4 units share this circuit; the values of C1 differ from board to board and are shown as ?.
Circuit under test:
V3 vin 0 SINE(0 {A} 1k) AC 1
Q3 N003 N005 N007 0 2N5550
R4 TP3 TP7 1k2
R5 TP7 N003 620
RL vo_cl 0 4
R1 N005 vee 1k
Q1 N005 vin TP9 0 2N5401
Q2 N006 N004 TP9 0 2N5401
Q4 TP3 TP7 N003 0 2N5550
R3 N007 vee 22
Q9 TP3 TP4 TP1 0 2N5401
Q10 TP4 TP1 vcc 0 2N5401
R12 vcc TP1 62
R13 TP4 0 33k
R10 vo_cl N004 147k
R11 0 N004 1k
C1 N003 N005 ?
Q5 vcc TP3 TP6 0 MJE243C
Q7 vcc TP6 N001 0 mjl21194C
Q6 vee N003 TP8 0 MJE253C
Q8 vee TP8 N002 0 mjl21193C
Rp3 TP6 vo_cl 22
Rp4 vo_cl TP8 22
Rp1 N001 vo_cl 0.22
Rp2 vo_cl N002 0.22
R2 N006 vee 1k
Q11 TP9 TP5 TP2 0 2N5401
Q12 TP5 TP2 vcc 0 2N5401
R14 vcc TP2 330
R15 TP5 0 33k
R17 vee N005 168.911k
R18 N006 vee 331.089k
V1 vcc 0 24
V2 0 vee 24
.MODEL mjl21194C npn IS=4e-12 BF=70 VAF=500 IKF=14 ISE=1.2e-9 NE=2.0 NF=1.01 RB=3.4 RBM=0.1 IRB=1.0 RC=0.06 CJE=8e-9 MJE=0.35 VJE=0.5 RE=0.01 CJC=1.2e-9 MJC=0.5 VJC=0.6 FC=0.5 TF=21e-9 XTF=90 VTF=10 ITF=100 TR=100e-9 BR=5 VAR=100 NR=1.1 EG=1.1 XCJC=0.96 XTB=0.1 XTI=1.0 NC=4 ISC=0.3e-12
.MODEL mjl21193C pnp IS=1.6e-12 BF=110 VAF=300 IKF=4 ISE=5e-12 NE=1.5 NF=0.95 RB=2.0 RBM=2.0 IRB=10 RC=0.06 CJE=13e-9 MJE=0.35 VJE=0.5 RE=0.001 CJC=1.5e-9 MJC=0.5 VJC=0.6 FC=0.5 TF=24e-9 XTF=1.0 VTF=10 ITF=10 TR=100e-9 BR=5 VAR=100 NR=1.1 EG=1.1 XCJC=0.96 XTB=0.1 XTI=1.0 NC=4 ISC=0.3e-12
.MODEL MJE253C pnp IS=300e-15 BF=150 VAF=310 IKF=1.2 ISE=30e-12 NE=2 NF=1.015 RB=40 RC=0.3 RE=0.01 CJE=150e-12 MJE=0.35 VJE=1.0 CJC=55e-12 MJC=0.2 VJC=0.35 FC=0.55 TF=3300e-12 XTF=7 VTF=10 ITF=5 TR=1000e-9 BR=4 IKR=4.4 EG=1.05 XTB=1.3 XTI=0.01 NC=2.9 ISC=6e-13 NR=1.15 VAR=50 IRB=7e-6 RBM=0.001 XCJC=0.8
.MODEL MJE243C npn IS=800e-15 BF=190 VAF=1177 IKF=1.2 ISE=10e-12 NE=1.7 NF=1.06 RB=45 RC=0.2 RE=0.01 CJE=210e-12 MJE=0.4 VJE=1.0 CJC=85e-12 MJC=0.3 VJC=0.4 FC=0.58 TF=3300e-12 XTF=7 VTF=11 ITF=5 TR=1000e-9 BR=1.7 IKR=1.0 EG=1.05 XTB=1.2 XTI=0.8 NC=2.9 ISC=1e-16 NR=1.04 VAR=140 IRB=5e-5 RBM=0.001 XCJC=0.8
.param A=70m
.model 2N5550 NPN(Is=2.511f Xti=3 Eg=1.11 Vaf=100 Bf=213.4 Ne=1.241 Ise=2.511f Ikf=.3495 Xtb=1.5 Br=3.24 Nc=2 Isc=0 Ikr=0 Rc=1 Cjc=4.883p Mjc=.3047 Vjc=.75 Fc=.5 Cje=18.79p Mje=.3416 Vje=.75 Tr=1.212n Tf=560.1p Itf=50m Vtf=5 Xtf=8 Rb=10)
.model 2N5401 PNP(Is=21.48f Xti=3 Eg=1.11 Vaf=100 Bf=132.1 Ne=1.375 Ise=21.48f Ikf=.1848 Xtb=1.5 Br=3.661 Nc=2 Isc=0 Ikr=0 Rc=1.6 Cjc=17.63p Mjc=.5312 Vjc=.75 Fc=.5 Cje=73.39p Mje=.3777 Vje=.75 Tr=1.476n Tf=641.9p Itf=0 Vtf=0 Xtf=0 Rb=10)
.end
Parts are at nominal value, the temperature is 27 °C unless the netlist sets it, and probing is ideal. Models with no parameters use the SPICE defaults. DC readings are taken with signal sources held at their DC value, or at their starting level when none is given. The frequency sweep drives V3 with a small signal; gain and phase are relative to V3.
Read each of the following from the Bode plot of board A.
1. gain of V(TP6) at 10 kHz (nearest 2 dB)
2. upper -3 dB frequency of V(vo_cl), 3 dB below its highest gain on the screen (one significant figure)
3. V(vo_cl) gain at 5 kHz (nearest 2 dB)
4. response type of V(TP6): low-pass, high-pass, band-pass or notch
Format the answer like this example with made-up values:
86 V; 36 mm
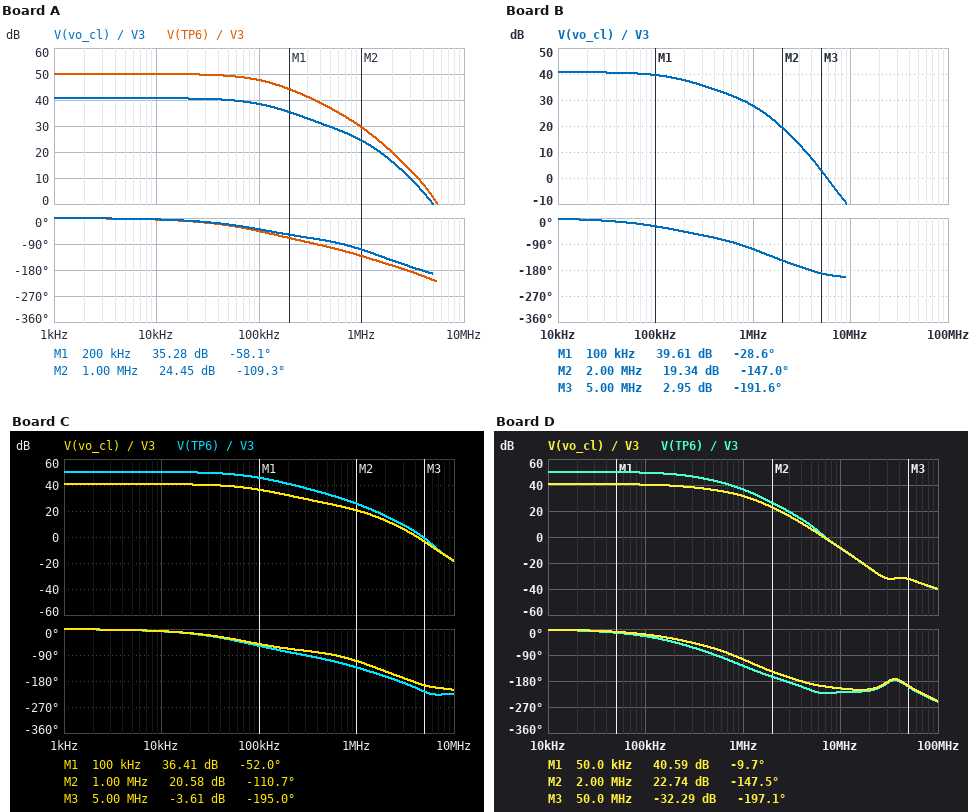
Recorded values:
50 dB; 100 kHz; 40 dB; low-pass
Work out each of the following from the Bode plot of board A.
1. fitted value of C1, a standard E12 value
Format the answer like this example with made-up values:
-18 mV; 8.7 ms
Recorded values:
47 pF
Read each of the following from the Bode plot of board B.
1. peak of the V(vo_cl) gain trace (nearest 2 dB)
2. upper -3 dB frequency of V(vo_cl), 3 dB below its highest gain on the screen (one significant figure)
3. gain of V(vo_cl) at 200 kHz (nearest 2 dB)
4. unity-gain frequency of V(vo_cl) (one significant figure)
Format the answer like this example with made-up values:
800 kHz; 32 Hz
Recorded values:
40 dB; 200 kHz; 38 dB; 6 MHz
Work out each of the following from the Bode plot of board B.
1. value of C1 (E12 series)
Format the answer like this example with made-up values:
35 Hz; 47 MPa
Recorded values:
27 pF
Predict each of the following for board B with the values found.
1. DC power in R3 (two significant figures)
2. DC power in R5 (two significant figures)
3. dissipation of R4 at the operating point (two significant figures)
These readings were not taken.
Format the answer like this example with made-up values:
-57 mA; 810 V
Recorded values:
2.2 mW; 900 µW; 2.0 mW
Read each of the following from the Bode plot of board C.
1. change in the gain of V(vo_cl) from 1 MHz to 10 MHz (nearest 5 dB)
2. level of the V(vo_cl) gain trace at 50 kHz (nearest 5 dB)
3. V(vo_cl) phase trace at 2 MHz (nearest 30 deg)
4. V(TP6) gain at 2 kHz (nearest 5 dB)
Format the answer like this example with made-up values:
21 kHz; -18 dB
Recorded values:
-40 dB; 40 dB; -150 deg; 50 dB
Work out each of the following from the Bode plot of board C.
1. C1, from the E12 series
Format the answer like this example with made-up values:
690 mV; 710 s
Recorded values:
82 pF
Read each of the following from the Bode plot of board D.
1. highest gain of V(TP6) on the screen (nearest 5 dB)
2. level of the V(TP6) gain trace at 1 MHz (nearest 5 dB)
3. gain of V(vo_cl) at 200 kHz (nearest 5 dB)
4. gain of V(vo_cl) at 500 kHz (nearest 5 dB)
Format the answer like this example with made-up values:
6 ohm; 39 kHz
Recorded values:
50 dB; 35 dB; 40 dB; 35 dB
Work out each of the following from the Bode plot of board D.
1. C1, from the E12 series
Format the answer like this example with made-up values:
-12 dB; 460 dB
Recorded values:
12 pF
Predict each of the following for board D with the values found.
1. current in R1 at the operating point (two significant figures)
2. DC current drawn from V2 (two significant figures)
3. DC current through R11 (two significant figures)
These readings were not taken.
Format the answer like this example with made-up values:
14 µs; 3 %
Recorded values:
970 µA; 34 mA; 6.0 µA
